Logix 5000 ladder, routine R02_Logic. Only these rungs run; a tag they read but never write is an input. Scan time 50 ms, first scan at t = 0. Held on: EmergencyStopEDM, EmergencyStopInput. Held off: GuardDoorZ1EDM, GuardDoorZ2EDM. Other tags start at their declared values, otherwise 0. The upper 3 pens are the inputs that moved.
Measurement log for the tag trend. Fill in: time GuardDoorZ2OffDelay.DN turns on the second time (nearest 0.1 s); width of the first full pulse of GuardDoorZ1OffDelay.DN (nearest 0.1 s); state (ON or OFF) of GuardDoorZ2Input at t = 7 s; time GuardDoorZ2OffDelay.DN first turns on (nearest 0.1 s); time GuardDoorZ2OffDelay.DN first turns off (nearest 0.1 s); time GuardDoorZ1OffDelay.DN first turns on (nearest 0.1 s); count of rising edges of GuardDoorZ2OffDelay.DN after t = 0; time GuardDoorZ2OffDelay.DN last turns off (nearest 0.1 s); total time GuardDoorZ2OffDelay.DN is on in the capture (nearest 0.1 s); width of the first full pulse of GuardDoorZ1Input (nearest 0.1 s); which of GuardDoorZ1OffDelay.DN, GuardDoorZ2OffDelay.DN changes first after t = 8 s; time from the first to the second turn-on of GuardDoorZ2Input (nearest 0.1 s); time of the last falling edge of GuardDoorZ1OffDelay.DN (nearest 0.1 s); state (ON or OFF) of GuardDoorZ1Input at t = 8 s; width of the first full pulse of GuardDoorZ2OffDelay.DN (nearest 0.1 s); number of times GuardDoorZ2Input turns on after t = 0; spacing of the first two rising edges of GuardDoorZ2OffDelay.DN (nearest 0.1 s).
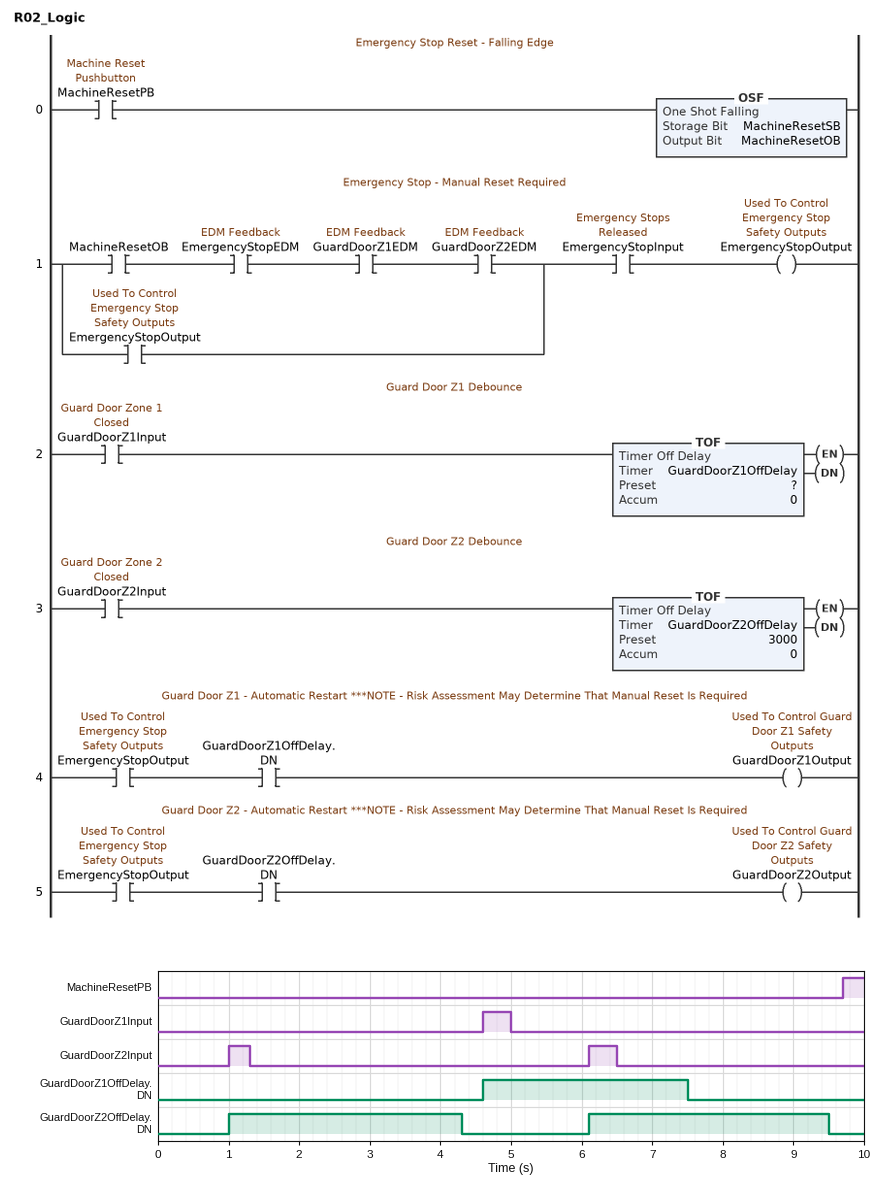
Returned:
6.1 s
2.9 s
OFF
1.0 s
4.3 s
4.6 s
2
9.5 s
6.7 s
0.4 s
GuardDoorZ2OffDelay.DN
5.1 s
7.5 s
OFF
3.3 s
2
5.1 s
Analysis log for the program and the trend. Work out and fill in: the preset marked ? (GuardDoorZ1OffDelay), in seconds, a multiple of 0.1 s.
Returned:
2.5 s
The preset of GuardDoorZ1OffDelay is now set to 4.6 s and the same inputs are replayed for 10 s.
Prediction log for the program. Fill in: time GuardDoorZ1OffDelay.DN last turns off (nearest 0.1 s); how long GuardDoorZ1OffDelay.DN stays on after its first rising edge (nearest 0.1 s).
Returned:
9.6 s
5.0 s
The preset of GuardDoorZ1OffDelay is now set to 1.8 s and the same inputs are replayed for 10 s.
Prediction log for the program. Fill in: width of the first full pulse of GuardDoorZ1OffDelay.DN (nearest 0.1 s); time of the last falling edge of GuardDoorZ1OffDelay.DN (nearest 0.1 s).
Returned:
2.2 s
6.8 s
